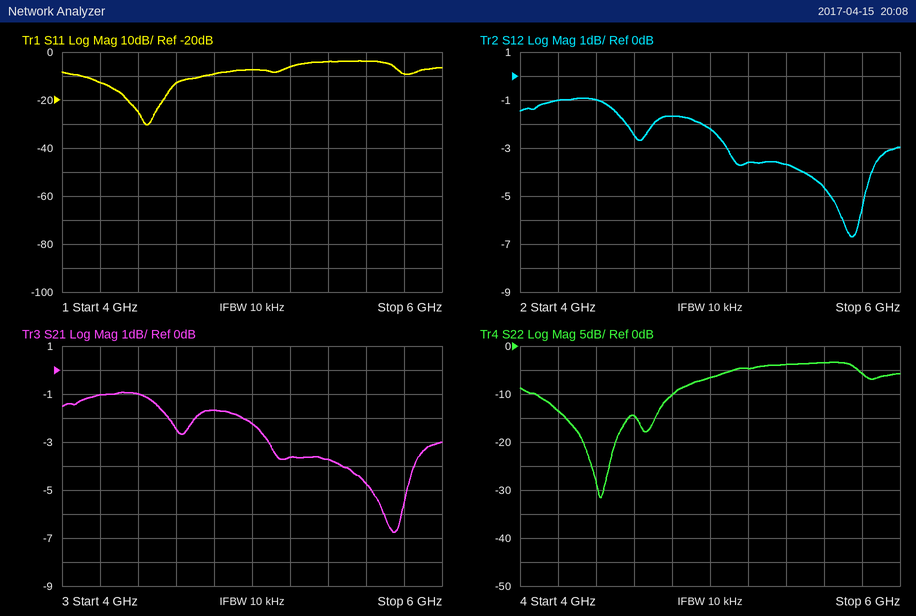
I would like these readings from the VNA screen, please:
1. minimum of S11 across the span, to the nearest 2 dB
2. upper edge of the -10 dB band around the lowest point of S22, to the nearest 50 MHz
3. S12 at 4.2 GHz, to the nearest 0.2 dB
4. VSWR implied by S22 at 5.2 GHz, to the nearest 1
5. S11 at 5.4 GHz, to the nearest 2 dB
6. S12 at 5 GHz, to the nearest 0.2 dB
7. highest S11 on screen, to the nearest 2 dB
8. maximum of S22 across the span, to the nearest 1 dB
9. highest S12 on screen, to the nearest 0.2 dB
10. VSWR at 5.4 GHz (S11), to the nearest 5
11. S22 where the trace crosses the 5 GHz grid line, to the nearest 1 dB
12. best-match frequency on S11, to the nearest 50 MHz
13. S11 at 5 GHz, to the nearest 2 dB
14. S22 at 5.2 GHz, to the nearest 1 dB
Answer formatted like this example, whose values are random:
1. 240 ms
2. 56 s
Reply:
1. -30 dB
2. 4.80 GHz
3. -1.0 dB
4. 4
5. -4 dB
6. -2.2 dB
7. -4 dB
8. -3 dB
9. -1.0 dB
10. 5
11. -7 dB
12. 4.45 GHz
13. -8 dB
14. -5 dB
